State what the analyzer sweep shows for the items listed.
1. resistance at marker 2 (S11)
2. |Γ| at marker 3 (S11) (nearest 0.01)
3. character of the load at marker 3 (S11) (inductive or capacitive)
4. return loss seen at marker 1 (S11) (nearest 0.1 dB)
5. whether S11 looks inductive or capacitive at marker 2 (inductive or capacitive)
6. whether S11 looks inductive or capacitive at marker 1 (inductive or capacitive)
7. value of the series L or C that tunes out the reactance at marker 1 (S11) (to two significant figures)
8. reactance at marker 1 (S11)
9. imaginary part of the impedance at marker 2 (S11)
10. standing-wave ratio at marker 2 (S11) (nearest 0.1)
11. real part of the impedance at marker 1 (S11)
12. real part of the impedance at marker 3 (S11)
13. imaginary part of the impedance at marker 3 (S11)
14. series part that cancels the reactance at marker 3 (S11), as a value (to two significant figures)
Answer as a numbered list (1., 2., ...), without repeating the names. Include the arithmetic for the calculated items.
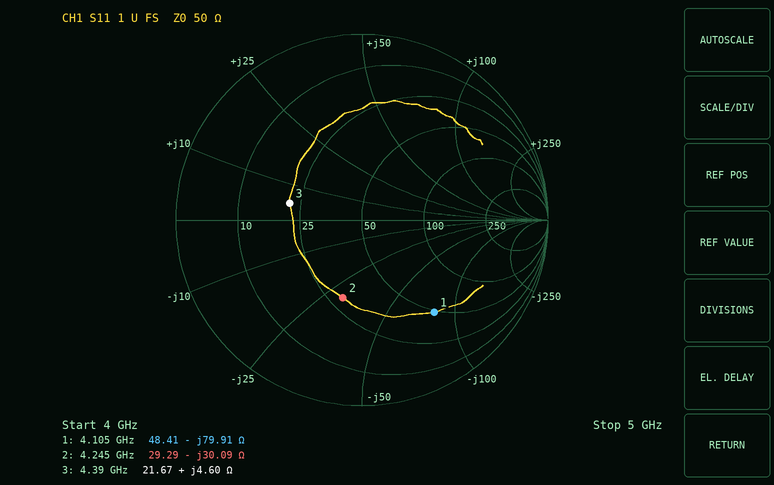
1. 29.29 Ω
2. 0.40
3. inductive
4. 4.0 dB
5. capacitive
6. capacitive
7. L = 79.91 Ω/(2π × 4.105 GHz) ≈ 3.1 nH
8. -79.91 Ω
9. -30.09 Ω
10. 2.5
11. 48.41 Ω
12. 21.67 Ω
13. +4.60 Ω
14. C = 1/(2π × 4.39 GHz × 4.6 Ω) ≈ 7.9 pF
